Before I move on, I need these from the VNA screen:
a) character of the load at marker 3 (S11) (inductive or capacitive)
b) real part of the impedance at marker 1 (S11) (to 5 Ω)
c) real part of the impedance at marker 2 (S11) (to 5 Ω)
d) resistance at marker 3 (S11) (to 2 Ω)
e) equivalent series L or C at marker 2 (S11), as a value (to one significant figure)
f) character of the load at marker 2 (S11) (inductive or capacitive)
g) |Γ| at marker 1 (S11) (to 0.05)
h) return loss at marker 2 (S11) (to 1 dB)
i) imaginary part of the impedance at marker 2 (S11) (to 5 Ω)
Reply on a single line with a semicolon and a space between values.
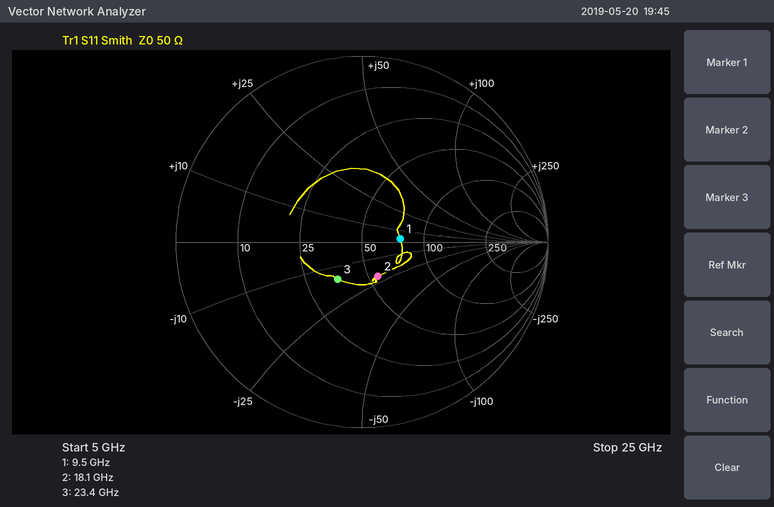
capacitive; 75 Ω; 55 Ω; 36 Ω; 400 fF; capacitive; 0.20; 14 dB; -20 Ω
